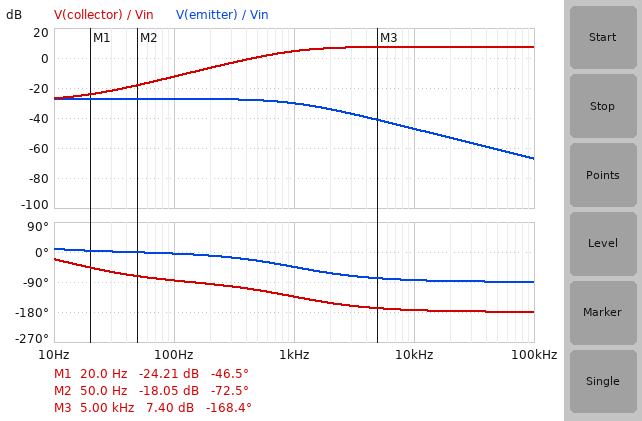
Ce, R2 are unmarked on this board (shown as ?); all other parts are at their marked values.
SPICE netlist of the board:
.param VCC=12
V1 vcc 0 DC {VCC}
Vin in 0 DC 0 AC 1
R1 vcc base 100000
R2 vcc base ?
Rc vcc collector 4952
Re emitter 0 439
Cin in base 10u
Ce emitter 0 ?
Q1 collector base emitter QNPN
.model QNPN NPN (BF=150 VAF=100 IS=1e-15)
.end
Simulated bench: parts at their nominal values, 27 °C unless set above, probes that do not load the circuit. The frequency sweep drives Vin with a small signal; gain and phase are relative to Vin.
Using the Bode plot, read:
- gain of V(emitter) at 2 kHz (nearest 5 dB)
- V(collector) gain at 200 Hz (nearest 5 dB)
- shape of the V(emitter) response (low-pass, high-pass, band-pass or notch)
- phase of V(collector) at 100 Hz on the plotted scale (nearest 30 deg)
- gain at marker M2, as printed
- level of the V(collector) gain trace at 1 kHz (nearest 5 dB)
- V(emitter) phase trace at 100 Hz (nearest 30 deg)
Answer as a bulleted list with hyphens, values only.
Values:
- -35 dB
- -5 dB
- low-pass
- -90 deg
- -18.05 dB
- 5 dB
- 0 deg
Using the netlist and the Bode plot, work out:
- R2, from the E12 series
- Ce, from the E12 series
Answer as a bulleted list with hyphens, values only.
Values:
- 27 kΩ
- 220 µF
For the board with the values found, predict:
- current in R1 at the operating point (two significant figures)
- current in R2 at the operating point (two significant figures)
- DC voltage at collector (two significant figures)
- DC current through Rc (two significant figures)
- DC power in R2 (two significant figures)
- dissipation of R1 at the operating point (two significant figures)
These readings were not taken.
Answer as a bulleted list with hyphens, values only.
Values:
- 100 µA
- 370 µA
- 1.2 V
- 2.2 mA
- 3.8 mW
- 1.0 mW
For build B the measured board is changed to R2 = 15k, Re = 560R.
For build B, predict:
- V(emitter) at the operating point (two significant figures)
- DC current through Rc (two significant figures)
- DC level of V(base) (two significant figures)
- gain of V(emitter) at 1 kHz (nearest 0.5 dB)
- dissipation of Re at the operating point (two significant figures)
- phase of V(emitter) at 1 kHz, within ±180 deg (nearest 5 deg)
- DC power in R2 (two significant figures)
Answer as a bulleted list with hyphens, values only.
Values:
- 1.6 V
- 2.1 mA
- 2.3 V
- -29.5 dB
- 4.5 mW
- -40 deg
- 6.2 mW
